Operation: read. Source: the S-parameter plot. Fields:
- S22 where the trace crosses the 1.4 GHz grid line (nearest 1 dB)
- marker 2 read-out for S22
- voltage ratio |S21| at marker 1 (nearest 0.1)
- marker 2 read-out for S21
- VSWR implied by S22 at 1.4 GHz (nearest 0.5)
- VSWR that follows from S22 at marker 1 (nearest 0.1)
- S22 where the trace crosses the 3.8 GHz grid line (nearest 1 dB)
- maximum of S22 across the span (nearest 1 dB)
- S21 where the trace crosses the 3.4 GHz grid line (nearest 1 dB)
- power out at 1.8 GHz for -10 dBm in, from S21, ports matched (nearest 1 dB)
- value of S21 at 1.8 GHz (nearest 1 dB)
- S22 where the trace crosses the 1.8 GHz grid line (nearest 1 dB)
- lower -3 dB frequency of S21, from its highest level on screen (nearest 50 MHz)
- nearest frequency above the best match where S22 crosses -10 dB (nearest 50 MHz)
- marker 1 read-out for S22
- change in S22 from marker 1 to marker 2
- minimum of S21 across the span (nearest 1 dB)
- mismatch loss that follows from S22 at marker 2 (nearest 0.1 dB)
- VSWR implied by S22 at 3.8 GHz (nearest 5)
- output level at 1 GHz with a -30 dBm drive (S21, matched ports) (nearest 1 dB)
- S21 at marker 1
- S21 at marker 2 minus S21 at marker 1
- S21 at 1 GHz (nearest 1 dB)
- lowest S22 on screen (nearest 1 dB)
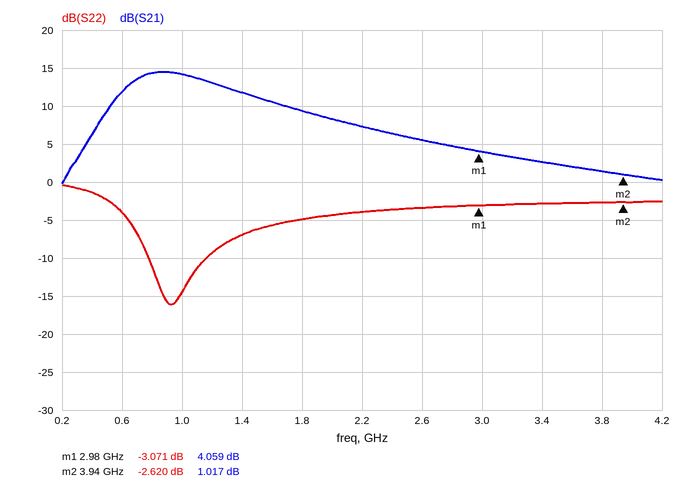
-7 dB
-2.620 dB
1.6
1.017 dB
2.5
5.7
-3 dB
0 dB
3 dB
-1 dBm
9 dB
-5 dB
600 MHz
1.15 GHz
-3.071 dB
0.451 dB
0 dB
3.4 dB
5
-16 dBm
4.059 dB
-3.042 dB
14 dB
-16 dB
